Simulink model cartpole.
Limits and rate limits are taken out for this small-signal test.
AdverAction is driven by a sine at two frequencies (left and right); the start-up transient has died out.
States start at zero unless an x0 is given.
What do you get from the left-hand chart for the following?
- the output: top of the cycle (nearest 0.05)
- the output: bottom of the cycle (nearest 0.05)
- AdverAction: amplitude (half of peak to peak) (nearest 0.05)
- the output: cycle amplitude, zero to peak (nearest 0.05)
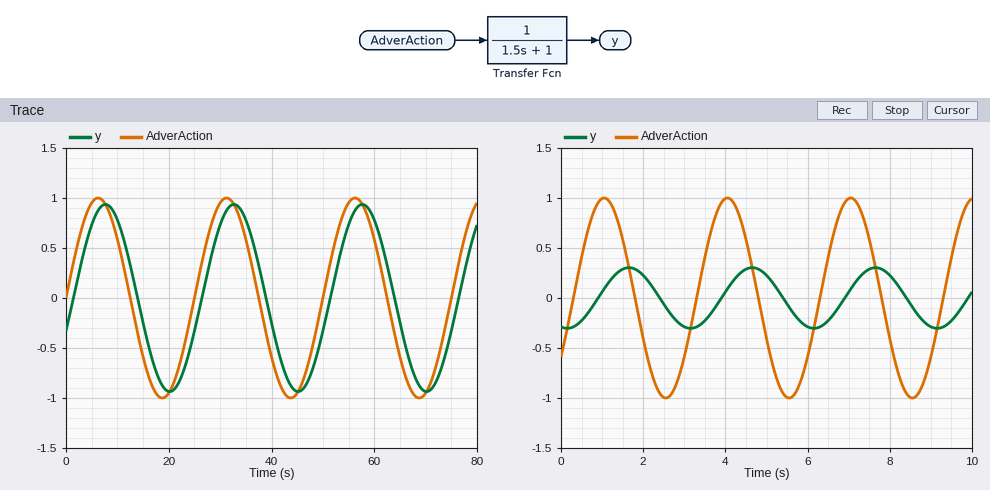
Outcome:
0.95
-0.95
1.00
0.95
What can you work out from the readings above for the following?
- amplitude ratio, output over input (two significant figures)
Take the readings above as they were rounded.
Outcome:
0.95
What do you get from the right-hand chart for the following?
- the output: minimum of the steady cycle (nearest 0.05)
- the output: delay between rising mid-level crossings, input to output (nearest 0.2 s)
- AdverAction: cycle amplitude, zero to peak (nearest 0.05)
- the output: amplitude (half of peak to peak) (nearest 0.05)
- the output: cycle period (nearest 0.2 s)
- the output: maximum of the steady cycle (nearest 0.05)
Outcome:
-0.30
0.6 s
1.00
0.30
3.0 s
0.30
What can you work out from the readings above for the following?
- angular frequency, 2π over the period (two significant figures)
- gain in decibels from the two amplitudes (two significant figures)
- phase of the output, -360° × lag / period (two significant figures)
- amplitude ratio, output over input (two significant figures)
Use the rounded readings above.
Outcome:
2.1 rad/s
-10 dB
-72°
0.30
